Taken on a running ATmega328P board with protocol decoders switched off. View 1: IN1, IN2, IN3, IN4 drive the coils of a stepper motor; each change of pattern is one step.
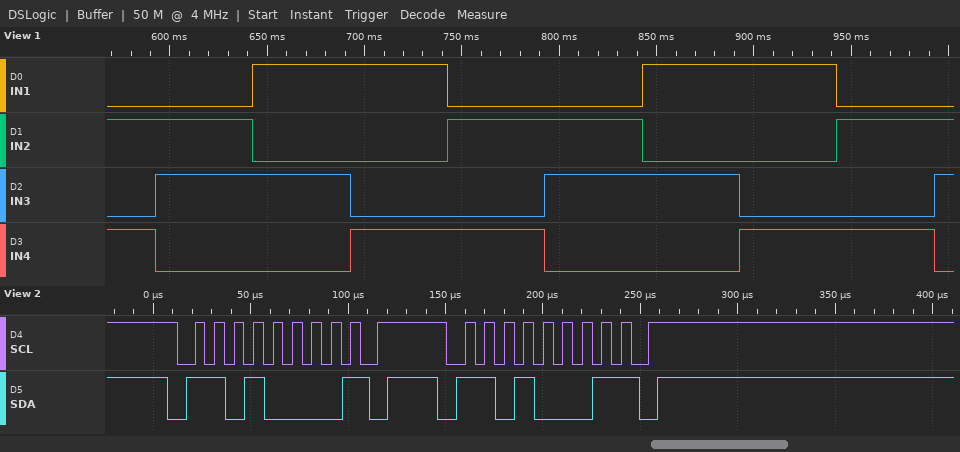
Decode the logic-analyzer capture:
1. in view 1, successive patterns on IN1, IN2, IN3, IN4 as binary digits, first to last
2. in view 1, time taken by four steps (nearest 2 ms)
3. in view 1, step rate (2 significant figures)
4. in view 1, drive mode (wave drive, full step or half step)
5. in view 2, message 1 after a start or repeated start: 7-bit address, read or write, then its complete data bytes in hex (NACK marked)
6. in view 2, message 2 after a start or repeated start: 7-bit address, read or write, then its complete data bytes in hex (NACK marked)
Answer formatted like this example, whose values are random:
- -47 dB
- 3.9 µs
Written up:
- 0101 0110 1010 1001 0101 0110 1010 1001 0101 0110
- 200 ms
- 20 steps/s
- full step
- 0x68 write NACK
- 0x68 read NACK
